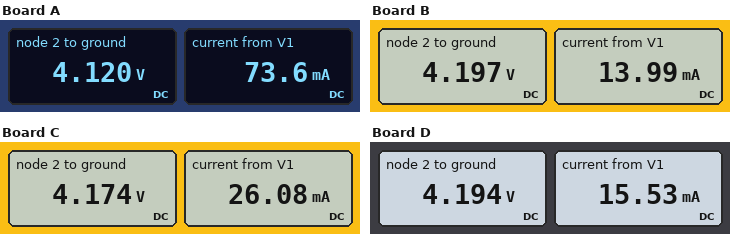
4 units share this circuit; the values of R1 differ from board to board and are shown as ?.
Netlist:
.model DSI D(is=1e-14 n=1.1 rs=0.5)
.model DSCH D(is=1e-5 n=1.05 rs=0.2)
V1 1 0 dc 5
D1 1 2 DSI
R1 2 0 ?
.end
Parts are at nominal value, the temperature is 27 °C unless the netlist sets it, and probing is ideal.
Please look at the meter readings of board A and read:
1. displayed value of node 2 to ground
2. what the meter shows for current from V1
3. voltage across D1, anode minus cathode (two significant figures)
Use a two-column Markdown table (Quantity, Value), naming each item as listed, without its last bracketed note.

| Quantity | Value |
|---|---|
| displayed value of node 2 to ground | 4.120 V |
| what the meter shows for current from V1 | 73.6 mA |
| voltage across D1, anode minus cathode | 880 mV |
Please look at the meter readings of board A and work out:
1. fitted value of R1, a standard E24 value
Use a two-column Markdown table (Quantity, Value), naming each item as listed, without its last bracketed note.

| Quantity | Value |
|---|---|
| fitted value of R1, a standard E24 value | 56 Ω |
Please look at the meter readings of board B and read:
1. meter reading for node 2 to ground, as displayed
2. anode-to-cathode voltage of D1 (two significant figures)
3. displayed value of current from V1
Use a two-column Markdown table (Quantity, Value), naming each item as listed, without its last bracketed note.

| Quantity | Value |
|---|---|
| meter reading for node 2 to ground, as displayed | 4.197 V |
| anode-to-cathode voltage of D1 | 800 mV |
| displayed value of current from V1 | 13.99 mA |
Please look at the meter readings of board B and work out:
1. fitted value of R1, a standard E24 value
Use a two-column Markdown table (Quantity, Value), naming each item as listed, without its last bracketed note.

| Quantity | Value |
|---|---|
| fitted value of R1, a standard E24 value | 300 Ω |
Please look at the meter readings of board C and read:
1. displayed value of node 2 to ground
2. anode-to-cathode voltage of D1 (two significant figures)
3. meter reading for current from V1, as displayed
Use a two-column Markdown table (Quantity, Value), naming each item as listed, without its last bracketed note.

| Quantity | Value |
|---|---|
| displayed value of node 2 to ground | 4.174 V |
| anode-to-cathode voltage of D1 | 830 mV |
| meter reading for current from V1, as displayed | 26.08 mA |
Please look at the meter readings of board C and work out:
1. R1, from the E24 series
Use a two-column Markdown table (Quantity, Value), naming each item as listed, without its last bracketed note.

| Quantity | Value |
|---|---|
| R1, from the E24 series | 160 Ω |
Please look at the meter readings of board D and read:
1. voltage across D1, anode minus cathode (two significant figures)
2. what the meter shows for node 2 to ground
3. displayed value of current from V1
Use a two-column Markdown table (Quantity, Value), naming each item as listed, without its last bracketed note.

| Quantity | Value |
|---|---|
| voltage across D1, anode minus cathode | 810 mV |
| what the meter shows for node 2 to ground | 4.194 V |
| displayed value of current from V1 | 15.53 mA |
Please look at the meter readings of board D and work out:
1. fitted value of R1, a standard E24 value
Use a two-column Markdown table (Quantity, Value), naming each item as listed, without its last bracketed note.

| Quantity | Value |
|---|---|
| fitted value of R1, a standard E24 value | 270 Ω |
